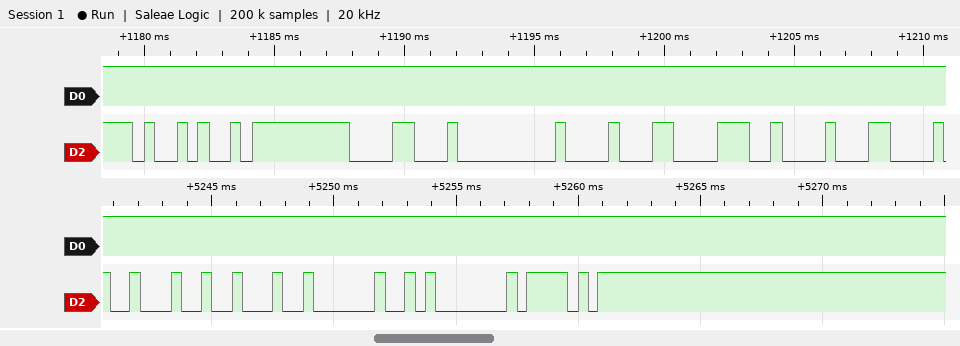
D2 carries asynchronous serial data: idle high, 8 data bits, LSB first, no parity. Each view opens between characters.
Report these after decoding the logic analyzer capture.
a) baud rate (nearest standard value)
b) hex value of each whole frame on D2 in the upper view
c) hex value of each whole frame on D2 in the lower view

2400 baud
29, FF, 18, 00, 88, 38, 88
22, 22, 20, 01, AF
